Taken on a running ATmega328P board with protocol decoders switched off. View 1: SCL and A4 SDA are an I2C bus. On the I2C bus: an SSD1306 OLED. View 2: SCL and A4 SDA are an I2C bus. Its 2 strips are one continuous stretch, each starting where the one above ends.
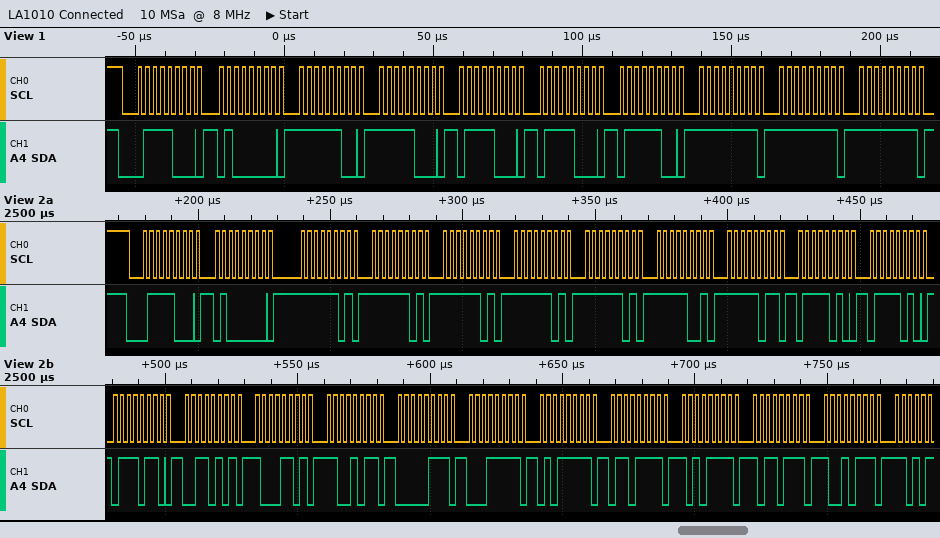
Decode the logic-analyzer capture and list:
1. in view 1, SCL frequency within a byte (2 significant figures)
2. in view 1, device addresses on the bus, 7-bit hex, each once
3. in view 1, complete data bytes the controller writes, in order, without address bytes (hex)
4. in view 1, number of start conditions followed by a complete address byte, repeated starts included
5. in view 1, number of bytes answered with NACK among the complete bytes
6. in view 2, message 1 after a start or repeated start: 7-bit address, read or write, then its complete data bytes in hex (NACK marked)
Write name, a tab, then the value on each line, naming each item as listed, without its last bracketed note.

in view 1, SCL frequency within a byte	400 kHz
in view 1, device addresses on the bus, 7-bit hex, each once	0x3C
in view 1, complete data bytes the controller writes, in order, without address bytes	40 FC F8 78 78 7C FF FF FF
in view 1, number of start conditions followed by a complete address byte, repeated starts included	1
in view 1, number of bytes answered with NACK among the complete bytes	0
in view 2, message 1 after a start or repeated start: 7-bit address, read or write, then its complete data bytes in hex	0x3C write: 40 FD FD FD FD FD F9 FB 7A 7A 76 35 8D CB 07 1F 5F 6F AF B7 97
